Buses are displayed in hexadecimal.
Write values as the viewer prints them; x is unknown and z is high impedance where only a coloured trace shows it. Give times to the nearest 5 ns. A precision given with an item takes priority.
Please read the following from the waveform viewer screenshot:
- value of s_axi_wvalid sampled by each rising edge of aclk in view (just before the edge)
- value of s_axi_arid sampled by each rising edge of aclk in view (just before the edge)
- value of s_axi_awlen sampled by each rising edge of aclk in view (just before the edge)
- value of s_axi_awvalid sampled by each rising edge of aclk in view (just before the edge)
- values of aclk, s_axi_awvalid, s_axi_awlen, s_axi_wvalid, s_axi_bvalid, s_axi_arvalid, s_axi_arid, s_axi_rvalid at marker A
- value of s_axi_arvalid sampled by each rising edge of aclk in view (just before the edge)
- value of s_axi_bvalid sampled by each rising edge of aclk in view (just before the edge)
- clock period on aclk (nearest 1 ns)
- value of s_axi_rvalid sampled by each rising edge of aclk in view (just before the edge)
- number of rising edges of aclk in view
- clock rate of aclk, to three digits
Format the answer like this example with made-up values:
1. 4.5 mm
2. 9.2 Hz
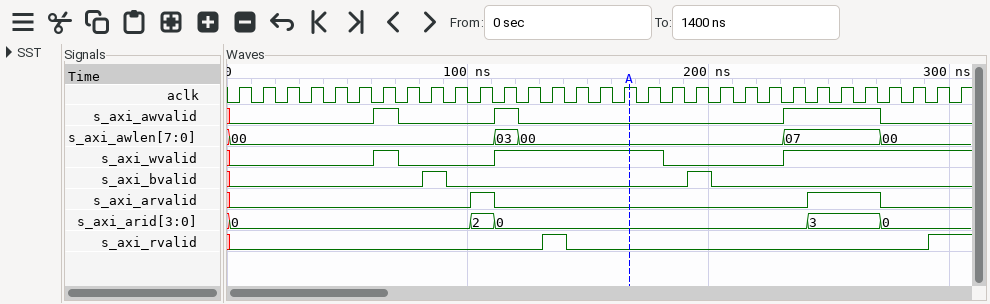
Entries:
1. 0 0 0 0 0 0 1 0 0 0 0 1 1 1 1 1 1 1 0 0 0 0 0 1 1 1 1 1 1 1 1
2. 0, 0, 0, 0, 0, 0, 0, 0, 0, 0, 2, 0, 0, 0, 0, 0, 0, 0, 0, 0, 0, 0, 0, 0, 3, 3, 3, 0, 0, 0, 0
3. 00, 00, 00, 00, 00, 00, 00, 00, 00, 00, 00, 03, 00, 00, 00, 00, 00, 00, 00, 00, 00, 00, 00, 07, 07, 07, 07, 00, 00, 00, 00
4. 0 0 0 0 0 0 1 0 0 0 0 1 0 0 0 0 0 0 0 0 0 0 0 1 1 1 1 0 0 0 0
5. aclk=1, s_axi_awvalid=0, s_axi_awlen=00, s_axi_wvalid=1, s_axi_bvalid=0, s_axi_arvalid=0, s_axi_arid=0, s_axi_rvalid=0
6. 0 0 0 0 0 0 0 0 0 0 1 0 0 0 0 0 0 0 0 0 0 0 0 0 1 1 1 0 0 0 0
7. 0 0 0 0 0 0 0 0 1 0 0 0 0 0 0 0 0 0 0 1 0 0 0 0 0 0 0 0 0 0 0
8. 10 ns
9. 0 0 0 0 0 0 0 0 0 0 0 0 0 1 0 0 0 0 0 0 0 0 0 0 0 0 0 0 0 1 1
10. 31
11. 100 MHz
